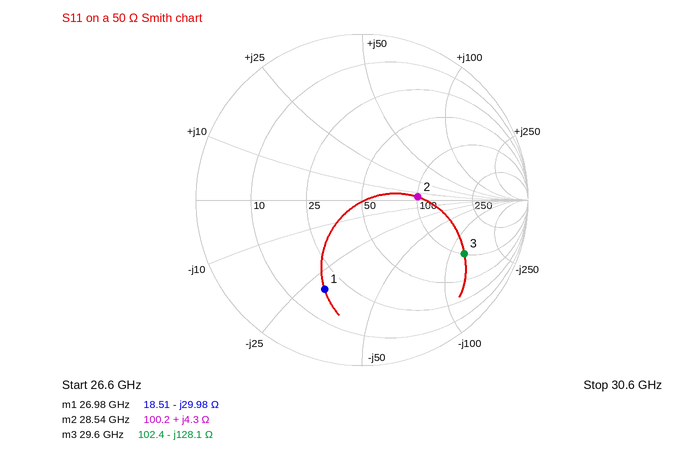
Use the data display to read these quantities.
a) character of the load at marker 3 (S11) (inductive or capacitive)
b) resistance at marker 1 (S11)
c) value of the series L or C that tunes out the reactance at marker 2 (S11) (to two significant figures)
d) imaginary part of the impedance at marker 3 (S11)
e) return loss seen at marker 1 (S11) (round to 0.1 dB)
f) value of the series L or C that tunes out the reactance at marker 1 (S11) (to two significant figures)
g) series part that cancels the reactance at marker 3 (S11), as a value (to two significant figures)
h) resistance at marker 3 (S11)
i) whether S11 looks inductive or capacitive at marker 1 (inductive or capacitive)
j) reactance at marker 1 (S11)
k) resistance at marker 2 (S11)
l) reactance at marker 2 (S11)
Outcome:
capacitive
18.51 Ω
1.3 pF
-128.1 Ω
4.7 dB
180 pH
690 pH
102.4 Ω
capacitive
-29.98 Ω
100.2 Ω
+4.3 Ω
